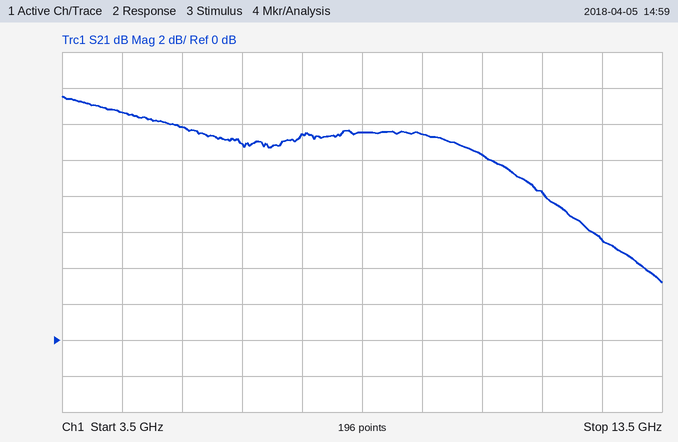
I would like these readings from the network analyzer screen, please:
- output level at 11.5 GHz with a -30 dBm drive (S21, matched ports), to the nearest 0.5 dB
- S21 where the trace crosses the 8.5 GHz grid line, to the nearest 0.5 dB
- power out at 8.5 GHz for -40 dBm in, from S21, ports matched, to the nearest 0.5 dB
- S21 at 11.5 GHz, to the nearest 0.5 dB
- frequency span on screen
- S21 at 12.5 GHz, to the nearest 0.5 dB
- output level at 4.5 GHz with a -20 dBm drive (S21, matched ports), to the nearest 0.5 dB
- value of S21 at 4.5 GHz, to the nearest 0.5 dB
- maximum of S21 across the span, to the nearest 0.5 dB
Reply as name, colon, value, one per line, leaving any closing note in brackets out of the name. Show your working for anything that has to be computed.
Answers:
output level at 11.5 GHz with a -30 dBm drive (S21, matched ports), to the nearest 0.5 dB: -30 dBm + (8.0 dB) = -22.0 dBm
S21 where the trace crosses the 8.5 GHz grid line, to the nearest 0.5 dB: 11.5 dB
power out at 8.5 GHz for -40 dBm in, from S21, ports matched, to the nearest 0.5 dB: -40 dBm + (11.5 dB) = -28.5 dBm
S21 at 11.5 GHz, to the nearest 0.5 dB: 8.0 dB
frequency span on screen: 10 GHz
S21 at 12.5 GHz, to the nearest 0.5 dB: 5.5 dB
output level at 4.5 GHz with a -20 dBm drive (S21, matched ports), to the nearest 0.5 dB: -20 dBm + (12.5 dB) = -7.5 dBm
value of S21 at 4.5 GHz, to the nearest 0.5 dB: 12.5 dB
maximum of S21 across the span, to the nearest 0.5 dB: 13.5 dB
